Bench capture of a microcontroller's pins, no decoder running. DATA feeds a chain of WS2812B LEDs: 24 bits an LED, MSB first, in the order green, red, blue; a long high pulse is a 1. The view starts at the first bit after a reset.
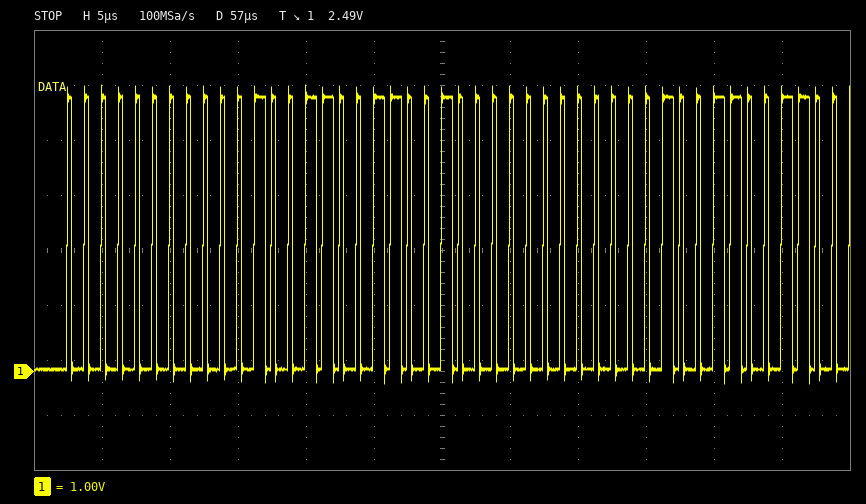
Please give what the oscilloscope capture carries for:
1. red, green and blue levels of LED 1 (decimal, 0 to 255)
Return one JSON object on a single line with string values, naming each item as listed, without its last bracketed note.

{"red, green and blue levels of LED 1": "19, 0, 50"}
